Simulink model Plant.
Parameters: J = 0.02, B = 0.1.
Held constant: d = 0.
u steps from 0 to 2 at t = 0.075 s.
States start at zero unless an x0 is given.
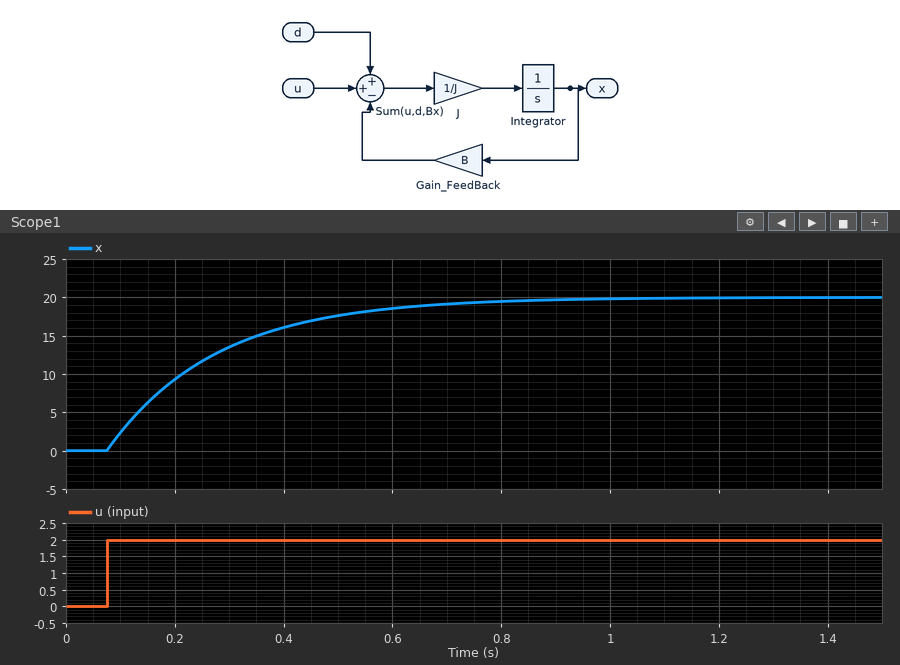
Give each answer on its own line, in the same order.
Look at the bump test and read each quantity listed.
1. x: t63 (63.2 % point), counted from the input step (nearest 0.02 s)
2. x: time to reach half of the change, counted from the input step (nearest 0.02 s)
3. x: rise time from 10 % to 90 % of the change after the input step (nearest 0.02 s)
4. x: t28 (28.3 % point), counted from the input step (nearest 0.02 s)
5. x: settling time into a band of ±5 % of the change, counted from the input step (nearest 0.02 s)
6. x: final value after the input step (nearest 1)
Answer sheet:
0.20 s
0.14 s
0.44 s
0.06 s
0.60 s
20
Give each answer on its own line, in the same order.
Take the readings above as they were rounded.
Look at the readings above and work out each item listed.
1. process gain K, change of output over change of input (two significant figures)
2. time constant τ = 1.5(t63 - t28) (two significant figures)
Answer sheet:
10
0.21 s
